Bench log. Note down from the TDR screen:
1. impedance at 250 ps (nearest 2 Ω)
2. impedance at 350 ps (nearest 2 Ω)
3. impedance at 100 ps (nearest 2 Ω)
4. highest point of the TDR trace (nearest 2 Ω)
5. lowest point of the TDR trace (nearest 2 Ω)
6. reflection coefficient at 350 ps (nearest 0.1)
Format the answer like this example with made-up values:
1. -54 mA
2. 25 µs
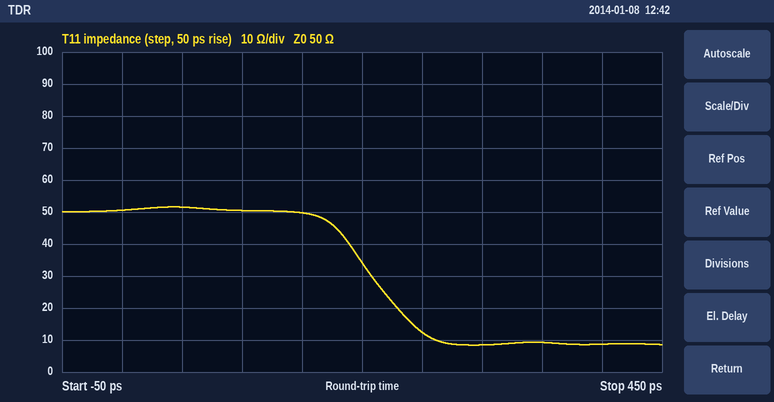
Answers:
1. 12 Ω
2. 10 Ω
3. 50 Ω
4. 52 Ω
5. 8 Ω
6. -0.7
